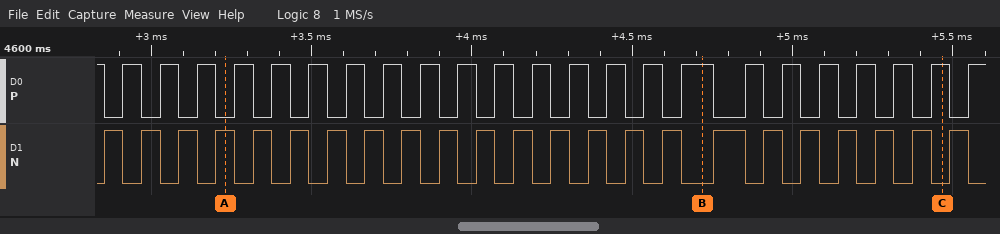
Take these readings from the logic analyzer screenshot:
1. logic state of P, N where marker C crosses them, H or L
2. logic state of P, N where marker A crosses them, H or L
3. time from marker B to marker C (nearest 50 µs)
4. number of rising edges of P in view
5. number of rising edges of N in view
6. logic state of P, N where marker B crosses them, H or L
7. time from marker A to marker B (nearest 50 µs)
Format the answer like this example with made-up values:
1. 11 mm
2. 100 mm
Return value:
1. P=H, N=L
2. P=L, N=H
3. 750 µs
4. 23
5. 23
6. P=H, N=L
7. 1500 µs
